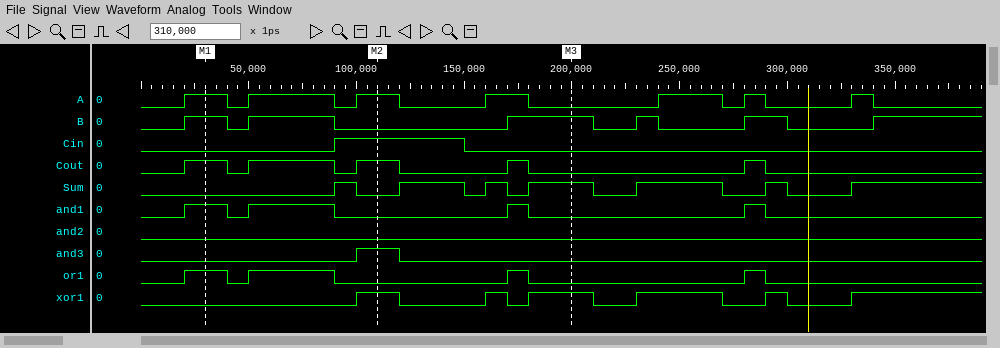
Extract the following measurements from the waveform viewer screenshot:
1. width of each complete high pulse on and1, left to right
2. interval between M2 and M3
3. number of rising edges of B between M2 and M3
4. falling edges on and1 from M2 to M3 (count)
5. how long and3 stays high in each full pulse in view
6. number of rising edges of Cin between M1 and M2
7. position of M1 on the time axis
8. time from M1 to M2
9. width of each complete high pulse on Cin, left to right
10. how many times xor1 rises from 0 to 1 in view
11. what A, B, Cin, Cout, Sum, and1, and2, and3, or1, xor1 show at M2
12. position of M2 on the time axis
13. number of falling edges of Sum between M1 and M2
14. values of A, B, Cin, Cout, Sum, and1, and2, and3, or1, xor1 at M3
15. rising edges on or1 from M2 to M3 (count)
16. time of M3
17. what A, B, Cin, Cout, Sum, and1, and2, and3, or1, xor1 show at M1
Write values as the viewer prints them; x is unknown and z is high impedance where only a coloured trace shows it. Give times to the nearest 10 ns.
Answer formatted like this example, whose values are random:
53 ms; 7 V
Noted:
20 ns, 40 ns, 10 ns, 10 ns; 90 ns; 1; 1; 20 ns; 1; 30 ns; 80 ns; 60 ns; 6; A=1, B=0, Cin=1, Cout=1, Sum=0, and1=0, and2=0, and3=1, or1=0, xor1=1; 110 ns; 1; A=0, B=1, Cin=0, Cout=0, Sum=1, and1=0, and2=0, and3=0, or1=0, xor1=1; 1; 200 ns; A=1, B=1, Cin=0, Cout=1, Sum=0, and1=1, and2=0, and3=0, or1=1, xor1=0
